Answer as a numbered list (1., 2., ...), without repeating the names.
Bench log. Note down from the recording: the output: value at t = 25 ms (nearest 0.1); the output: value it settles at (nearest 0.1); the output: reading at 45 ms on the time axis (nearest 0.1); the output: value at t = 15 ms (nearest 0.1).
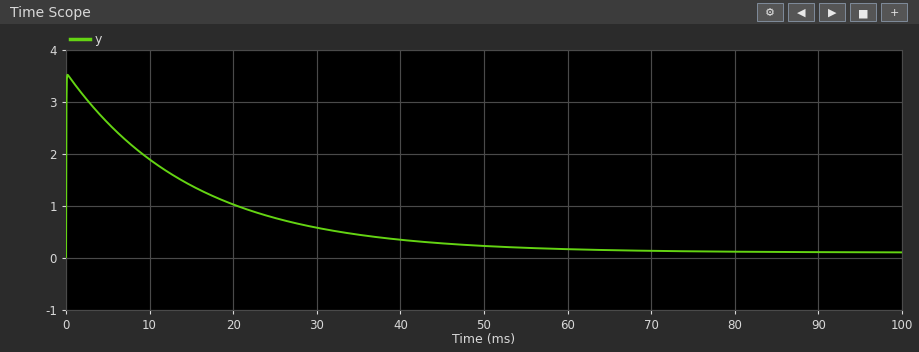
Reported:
1. 0.8
2. 0.1
3. 0.3
4. 1.4
